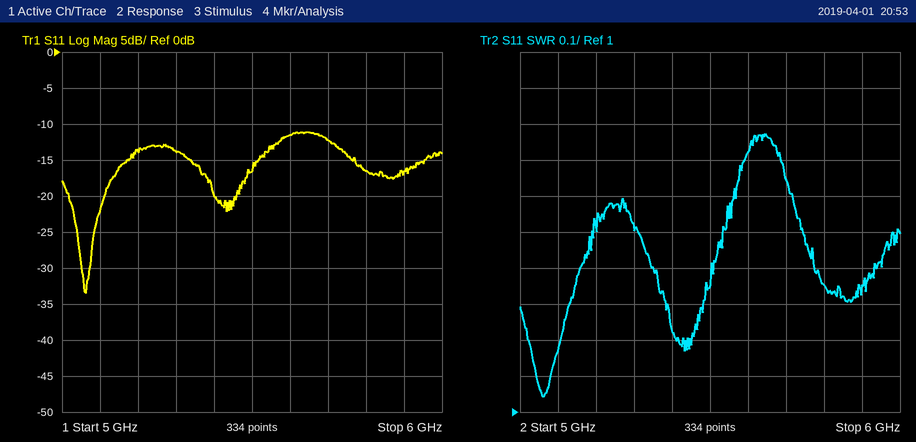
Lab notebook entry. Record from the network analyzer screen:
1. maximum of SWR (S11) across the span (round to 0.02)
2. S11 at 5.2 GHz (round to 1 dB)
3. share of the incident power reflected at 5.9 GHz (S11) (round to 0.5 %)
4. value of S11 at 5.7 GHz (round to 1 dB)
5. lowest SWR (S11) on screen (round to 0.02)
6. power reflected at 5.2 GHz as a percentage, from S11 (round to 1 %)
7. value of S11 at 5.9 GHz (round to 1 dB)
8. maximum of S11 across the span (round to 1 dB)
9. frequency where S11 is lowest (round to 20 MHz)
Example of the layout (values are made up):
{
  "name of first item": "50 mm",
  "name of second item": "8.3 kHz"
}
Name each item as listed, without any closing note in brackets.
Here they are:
{
  "maximum of SWR (S11) across the span": "1.78",
  "S11 at 5.2 GHz": "-14 dB",
  "share of the incident power reflected at 5.9 GHz (S11)": "2.0 %",
  "value of S11 at 5.7 GHz": "-12 dB",
  "lowest SWR (S11) on screen": "1.04",
  "power reflected at 5.2 GHz as a percentage, from S11": "4 %",
  "value of S11 at 5.9 GHz": "-17 dB",
  "maximum of S11 across the span": "-11 dB",
  "frequency where S11 is lowest": "5.06 GHz"
}
